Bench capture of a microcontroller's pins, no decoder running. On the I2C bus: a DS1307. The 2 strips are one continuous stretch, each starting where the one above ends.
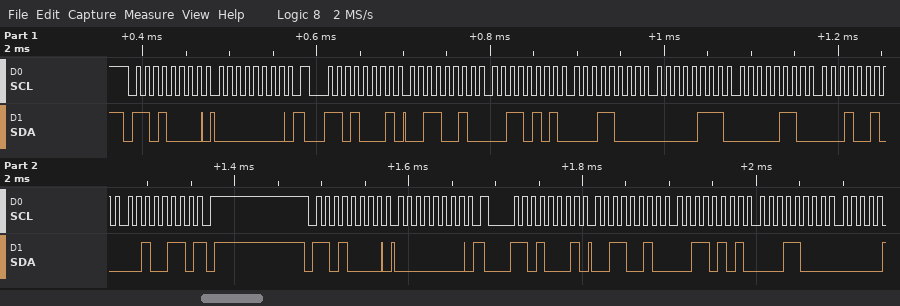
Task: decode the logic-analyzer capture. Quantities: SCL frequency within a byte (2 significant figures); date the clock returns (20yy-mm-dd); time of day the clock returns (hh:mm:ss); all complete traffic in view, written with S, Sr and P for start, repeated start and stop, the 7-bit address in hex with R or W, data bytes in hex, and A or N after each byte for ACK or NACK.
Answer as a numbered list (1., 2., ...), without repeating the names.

1. 100 kHz
2. 2026-12-06
3. 18:35:32
4. S 68W A 00 A Sr 68R A 32 A 35 A 18 A 07 A 06 A 12 A 26 N P S 68W A 00 A Sr 68R A 32 A 35 A 18 A
